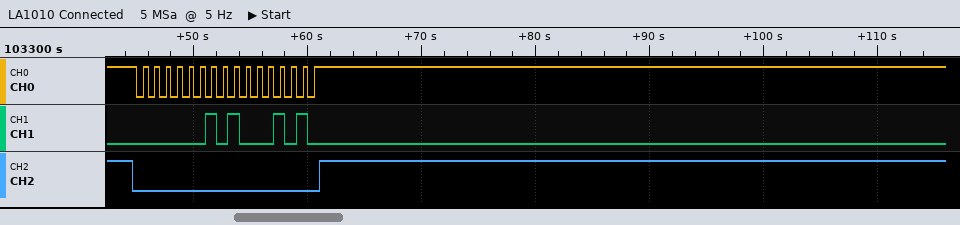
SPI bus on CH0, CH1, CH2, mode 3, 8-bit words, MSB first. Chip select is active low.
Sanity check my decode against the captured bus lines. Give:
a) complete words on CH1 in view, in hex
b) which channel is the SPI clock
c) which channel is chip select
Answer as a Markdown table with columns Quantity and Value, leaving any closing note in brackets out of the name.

| Quantity | Value |
|---|---|
| complete words on CH1 in view, in hex | 02, 8A |
| which channel is the SPI clock | CH0 |
| which channel is chip select | CH2 |
